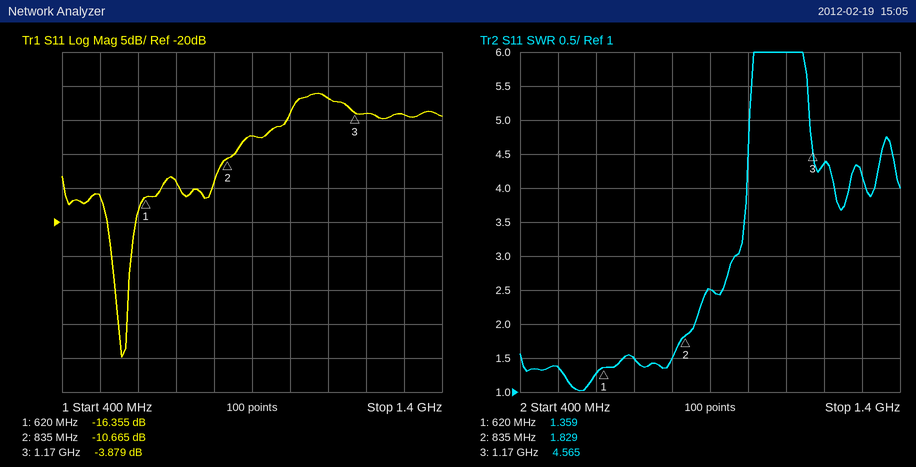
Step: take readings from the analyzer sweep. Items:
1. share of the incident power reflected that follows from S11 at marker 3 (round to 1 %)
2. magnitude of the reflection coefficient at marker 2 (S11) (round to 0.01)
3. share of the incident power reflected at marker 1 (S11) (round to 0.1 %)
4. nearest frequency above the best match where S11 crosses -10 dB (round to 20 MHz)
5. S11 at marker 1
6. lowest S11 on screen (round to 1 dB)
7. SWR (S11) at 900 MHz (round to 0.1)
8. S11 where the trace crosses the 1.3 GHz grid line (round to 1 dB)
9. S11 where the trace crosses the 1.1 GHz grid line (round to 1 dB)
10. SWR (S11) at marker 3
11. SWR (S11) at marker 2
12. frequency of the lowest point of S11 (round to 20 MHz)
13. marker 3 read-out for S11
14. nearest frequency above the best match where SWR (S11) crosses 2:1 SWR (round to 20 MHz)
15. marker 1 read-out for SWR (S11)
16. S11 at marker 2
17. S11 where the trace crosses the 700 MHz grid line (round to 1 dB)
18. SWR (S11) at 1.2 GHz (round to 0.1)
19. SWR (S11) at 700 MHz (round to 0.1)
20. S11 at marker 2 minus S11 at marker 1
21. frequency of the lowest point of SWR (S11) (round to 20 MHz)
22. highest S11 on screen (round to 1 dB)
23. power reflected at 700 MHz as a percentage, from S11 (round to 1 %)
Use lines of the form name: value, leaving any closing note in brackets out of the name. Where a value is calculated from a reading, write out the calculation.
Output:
share of the incident power reflected that follows from S11 at marker 3: 10^(-3.879/10) ≈ 41 %
magnitude of the reflection coefficient at marker 2 (S11): 10^(-10.665/20) ≈ 0.29
share of the incident power reflected at marker 1 (S11): 10^(-16.355/10) ≈ 2.3 %
nearest frequency above the best match where S11 crosses -10 dB: 860 MHz
S11 at marker 1: -16.355 dB
lowest S11 on screen: -40 dB
SWR (S11) at 900 MHz: 2.5
S11 where the trace crosses the 1.3 GHz grid line: -4 dB
S11 where the trace crosses the 1.1 GHz grid line: -2 dB
SWR (S11) at marker 3: 4.565
SWR (S11) at marker 2: 1.829
frequency of the lowest point of S11: 560 MHz
marker 3 read-out for S11: -3.879 dB
nearest frequency above the best match where SWR (S11) crosses 2:1 SWR: 860 MHz
marker 1 read-out for SWR: 1.359
S11 at marker 2: -10.665 dB
S11 where the trace crosses the 700 MHz grid line: -14 dB
SWR (S11) at 1.2 GHz: 4.4
SWR (S11) at 700 MHz: 1.5
S11 at marker 2 minus S11 at marker 1: -10.665 − (-16.355) = 5.690 dB
frequency of the lowest point of SWR (S11): 560 MHz
highest S11 on screen: -1 dB
power reflected at 700 MHz as a percentage, from S11: 10^(-14/10) ≈ 4 %
